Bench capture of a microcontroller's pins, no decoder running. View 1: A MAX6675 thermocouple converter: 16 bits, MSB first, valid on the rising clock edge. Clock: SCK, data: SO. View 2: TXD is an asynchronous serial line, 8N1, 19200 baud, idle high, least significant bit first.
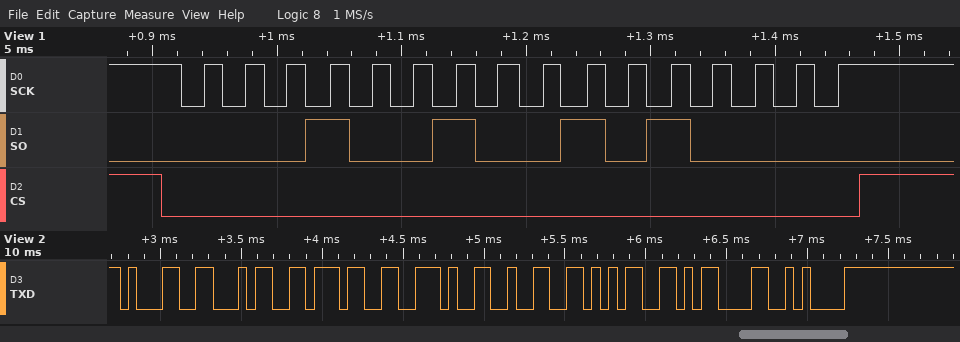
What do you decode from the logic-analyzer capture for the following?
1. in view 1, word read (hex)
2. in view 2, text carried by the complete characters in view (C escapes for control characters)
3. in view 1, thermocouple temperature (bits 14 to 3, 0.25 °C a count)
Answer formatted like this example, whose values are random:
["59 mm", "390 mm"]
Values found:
["0x1250", "\"147.25\\r\\n\"", "146.50 °C"]
